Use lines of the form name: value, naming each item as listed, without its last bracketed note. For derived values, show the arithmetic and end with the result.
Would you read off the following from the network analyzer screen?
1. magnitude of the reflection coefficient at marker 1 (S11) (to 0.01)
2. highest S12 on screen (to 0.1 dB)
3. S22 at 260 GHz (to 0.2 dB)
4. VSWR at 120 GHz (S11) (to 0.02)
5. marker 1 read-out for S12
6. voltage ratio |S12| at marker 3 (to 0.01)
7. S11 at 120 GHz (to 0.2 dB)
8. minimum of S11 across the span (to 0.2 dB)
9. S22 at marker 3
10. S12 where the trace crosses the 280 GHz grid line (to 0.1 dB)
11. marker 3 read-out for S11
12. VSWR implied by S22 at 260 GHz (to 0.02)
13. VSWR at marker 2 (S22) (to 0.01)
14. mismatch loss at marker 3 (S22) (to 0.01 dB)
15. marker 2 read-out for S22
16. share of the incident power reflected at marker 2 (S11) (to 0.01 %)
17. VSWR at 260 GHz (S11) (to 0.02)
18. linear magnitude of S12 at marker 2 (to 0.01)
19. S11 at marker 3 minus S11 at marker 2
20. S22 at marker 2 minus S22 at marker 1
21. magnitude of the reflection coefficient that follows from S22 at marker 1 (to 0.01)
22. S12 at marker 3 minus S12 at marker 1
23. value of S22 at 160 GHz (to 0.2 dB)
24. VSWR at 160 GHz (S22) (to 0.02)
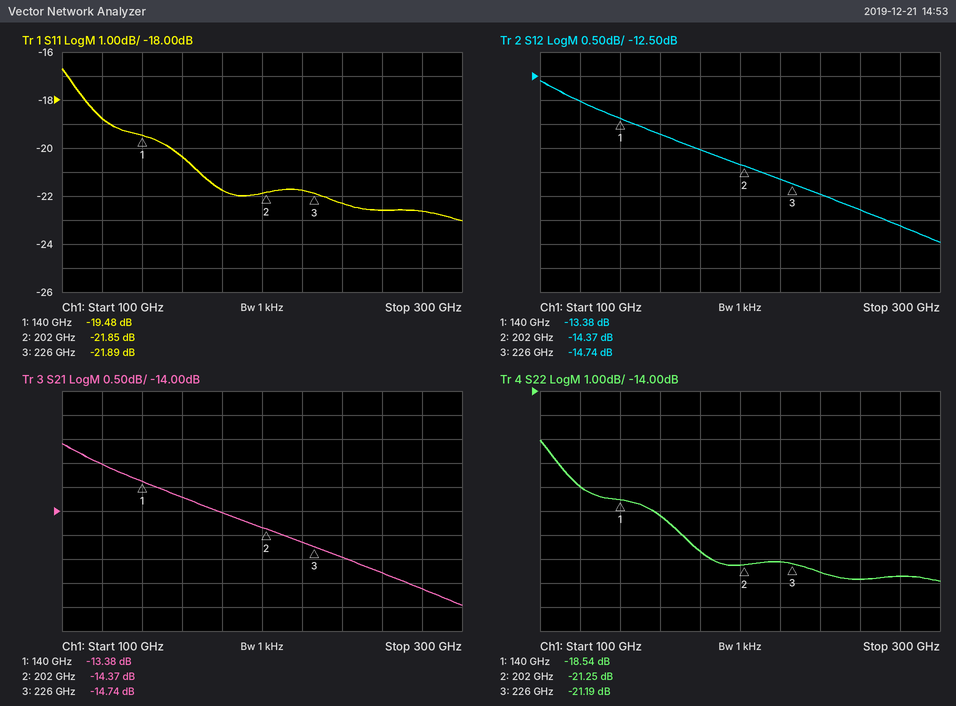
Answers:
magnitude of the reflection coefficient at marker 1 (S11): 10^(-19.48/20) ≈ 0.11
highest S12 on screen: -12.6 dB
S22 at 260 GHz: -21.8 dB
VSWR at 120 GHz (S11): |Γ| = 10^(-18.8/20) = 0.1148; VSWR = (1 + 0.1148)/(1 − 0.1148) ≈ 1.26
marker 1 read-out for S12: -13.38 dB
voltage ratio |S12| at marker 3: 10^(-14.74/20) ≈ 0.18
S11 at 120 GHz: -18.8 dB
minimum of S11 across the span: -23.0 dB
S22 at marker 3: -21.19 dB
S12 where the trace crosses the 280 GHz grid line: -15.6 dB
marker 3 read-out for S11: -21.89 dB
VSWR implied by S22 at 260 GHz: |Γ| = 10^(-21.8/20) = 0.0813; VSWR = (1 + 0.0813)/(1 − 0.0813) ≈ 1.18
VSWR at marker 2 (S22): (1 + 0.0866)/(1 − 0.0866) ≈ 1.19
mismatch loss at marker 3 (S22): −10 log10(1 − 10^(-21.19/10)) ≈ 0.03 dB
marker 2 read-out for S22: -21.25 dB
share of the incident power reflected at marker 2 (S11): 10^(-21.85/10) ≈ 0.65 %
VSWR at 260 GHz (S11): |Γ| = 10^(-22.6/20) = 0.0741; VSWR = (1 + 0.0741)/(1 − 0.0741) ≈ 1.16
linear magnitude of S12 at marker 2: 10^(-14.37/20) ≈ 0.19
S11 at marker 3 minus S11 at marker 2: -21.89 − (-21.85) = -0.04 dB
S22 at marker 2 minus S22 at marker 1: -21.25 − (-18.54) = -2.71 dB
magnitude of the reflection coefficient that follows from S22 at marker 1: 10^(-18.54/20) ≈ 0.12
S12 at marker 3 minus S12 at marker 1: -14.74 − (-13.38) = -1.36 dB
value of S22 at 160 GHz: -19.2 dB
VSWR at 160 GHz (S22): |Γ| = 10^(-19.2/20) = 0.1096; VSWR = (1 + 0.1096)/(1 − 0.1096) ≈ 1.25, so 1.24 to the nearest 0.02
